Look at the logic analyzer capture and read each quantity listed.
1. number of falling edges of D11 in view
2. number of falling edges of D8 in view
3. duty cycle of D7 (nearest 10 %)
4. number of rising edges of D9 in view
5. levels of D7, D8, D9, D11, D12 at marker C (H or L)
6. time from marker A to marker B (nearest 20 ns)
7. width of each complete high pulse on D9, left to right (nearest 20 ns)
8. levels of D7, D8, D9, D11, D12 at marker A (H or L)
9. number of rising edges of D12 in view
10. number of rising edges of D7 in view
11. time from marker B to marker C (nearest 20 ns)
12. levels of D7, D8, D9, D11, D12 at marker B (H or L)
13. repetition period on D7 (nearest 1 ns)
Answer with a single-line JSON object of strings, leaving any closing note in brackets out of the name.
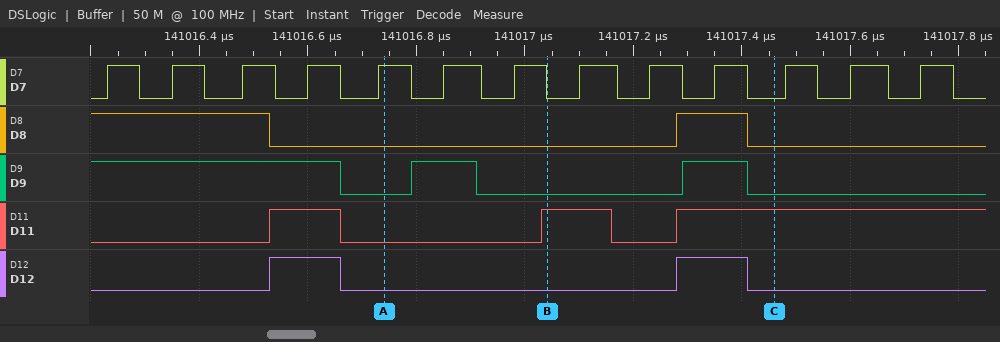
{"number of falling edges of D11 in view": "2", "number of falling edges of D8 in view": "2", "duty cycle of D7": "50 %", "number of rising edges of D9 in view": "2", "levels of D7, D8, D9, D11, D12 at marker C": "D7=L, D8=L, D9=L, D11=H, D12=L", "time from marker A to marker B": "300 ns", "width of each complete high pulse on D9, left to right": "120 ns, 120 ns", "levels of D7, D8, D9, D11, D12 at marker A": "D7=H, D8=L, D9=L, D11=L, D12=L", "number of rising edges of D12 in view": "2", "number of rising edges of D7 in view": "13", "time from marker B to marker C": "420 ns", "levels of D7, D8, D9, D11, D12 at marker B": "D7=L, D8=L, D9=L, D11=H, D12=L", "repetition period on D7": "125 ns"}
